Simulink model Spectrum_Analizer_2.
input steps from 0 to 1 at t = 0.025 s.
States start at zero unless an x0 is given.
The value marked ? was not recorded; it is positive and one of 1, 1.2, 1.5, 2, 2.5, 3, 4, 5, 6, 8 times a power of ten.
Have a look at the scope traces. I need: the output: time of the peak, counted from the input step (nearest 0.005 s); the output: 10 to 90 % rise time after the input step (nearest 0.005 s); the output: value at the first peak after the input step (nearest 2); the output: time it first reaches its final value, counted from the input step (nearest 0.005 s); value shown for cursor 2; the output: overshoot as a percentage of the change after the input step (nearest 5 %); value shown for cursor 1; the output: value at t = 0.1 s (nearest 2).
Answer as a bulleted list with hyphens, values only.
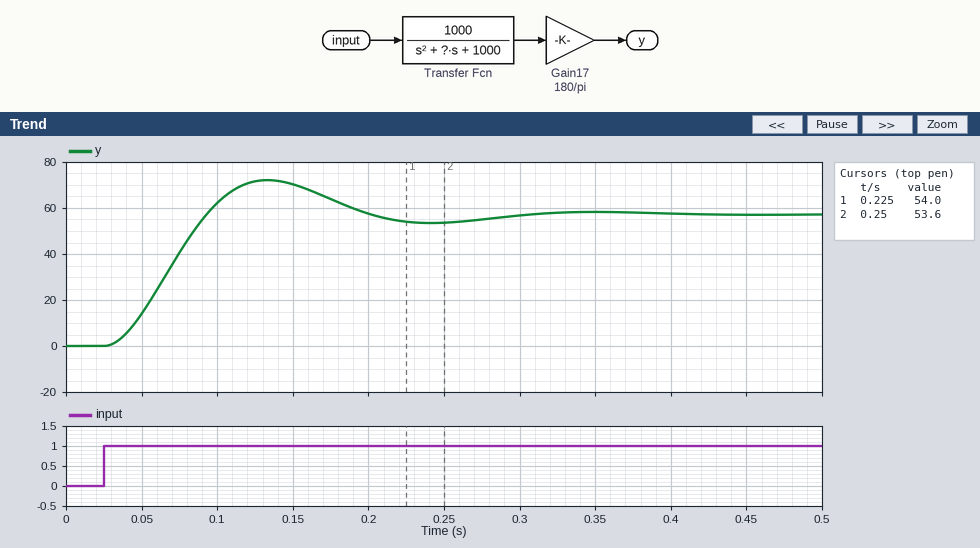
- 0.110 s
- 0.045 s
- 72
- 0.070 s
- 53.6
- 25 %
- 54.0
- 62
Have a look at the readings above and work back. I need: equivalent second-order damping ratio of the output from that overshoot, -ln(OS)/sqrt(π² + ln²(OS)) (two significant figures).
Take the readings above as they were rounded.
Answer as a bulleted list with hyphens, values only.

- 0.40
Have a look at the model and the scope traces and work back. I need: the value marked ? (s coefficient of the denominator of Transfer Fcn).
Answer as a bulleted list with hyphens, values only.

- 25
